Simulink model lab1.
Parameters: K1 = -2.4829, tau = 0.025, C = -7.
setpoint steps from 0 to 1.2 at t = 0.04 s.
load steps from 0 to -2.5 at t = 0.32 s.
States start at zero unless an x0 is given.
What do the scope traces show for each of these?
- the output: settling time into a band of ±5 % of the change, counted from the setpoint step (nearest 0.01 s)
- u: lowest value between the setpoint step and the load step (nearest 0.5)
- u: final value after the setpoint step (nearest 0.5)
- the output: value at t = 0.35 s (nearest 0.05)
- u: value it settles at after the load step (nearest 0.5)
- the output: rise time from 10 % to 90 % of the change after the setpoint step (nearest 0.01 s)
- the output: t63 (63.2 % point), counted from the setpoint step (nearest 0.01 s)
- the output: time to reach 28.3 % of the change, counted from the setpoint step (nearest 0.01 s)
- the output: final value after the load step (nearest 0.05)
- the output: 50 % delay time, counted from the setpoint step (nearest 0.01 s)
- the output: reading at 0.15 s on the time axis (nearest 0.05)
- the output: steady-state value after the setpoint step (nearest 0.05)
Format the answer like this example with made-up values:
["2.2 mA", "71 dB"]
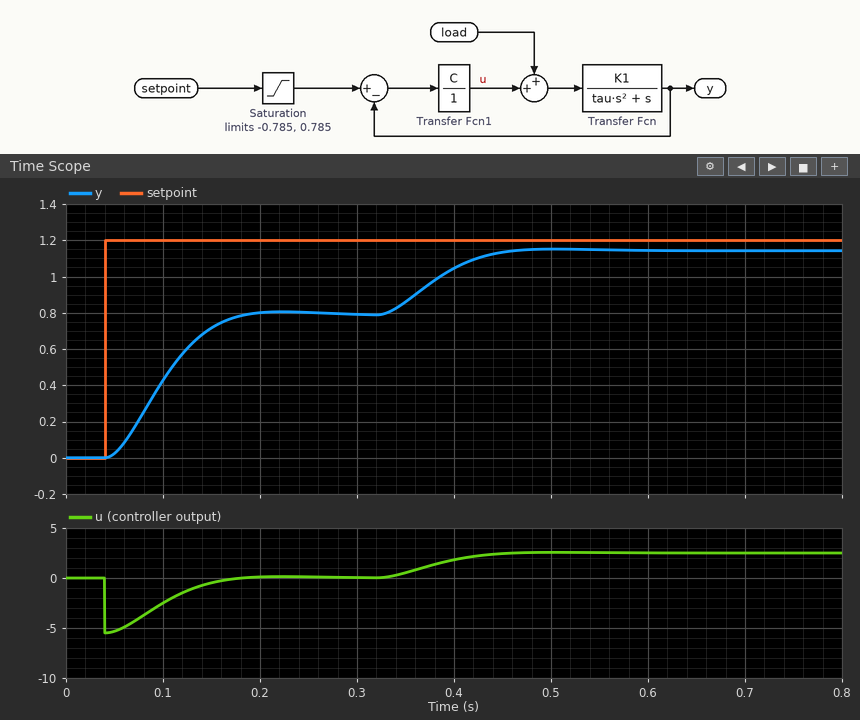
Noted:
["0.12 s", "-5.5", "0.0", "0.85", "2.5", "0.09 s", "0.07 s", "0.04 s", "1.15", "0.06 s", "0.70", "0.80"]
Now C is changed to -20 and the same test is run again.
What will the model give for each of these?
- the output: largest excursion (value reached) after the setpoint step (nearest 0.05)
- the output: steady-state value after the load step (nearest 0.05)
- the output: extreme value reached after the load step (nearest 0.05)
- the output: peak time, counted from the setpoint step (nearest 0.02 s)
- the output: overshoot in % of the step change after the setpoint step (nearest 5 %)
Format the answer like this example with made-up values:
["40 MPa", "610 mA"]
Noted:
["0.95", "0.90", "0.95", "0.08 s", "20 %"]
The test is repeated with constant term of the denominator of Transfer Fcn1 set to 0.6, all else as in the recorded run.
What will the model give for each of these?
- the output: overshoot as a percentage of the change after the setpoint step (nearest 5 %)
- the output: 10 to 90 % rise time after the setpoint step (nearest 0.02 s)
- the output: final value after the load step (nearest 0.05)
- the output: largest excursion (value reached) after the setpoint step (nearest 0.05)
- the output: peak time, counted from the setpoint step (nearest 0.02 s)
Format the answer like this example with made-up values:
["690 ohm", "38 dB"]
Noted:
["10 %", "0.06 s", "1.00", "0.85", "0.12 s"]
